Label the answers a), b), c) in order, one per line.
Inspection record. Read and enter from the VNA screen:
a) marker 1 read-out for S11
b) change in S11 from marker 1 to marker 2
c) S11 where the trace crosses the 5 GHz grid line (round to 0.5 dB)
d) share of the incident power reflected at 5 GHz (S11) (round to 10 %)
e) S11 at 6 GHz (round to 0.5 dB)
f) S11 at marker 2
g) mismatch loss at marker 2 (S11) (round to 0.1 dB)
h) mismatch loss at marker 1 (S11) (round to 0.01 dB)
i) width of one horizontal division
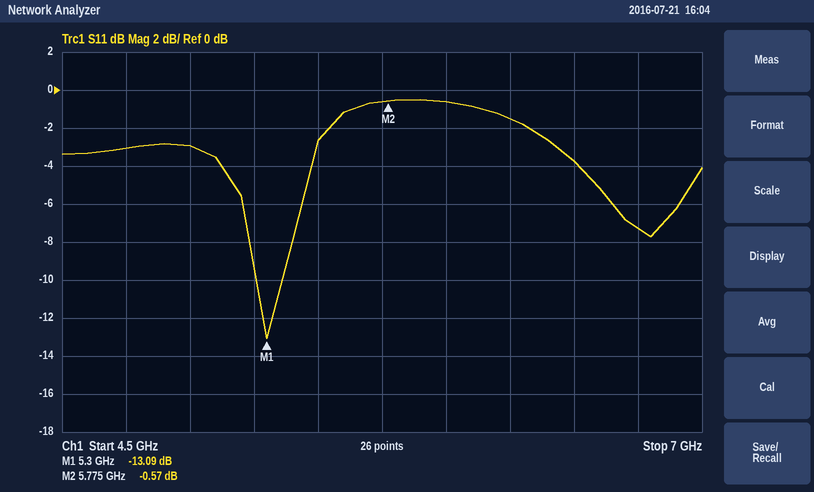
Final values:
a) -13.09 dB
b) 12.52 dB
c) -3.0 dB
d) 50 %
e) -0.5 dB
f) -0.57 dB
g) 9.1 dB
h) 0.22 dB
i) 250 MHz
